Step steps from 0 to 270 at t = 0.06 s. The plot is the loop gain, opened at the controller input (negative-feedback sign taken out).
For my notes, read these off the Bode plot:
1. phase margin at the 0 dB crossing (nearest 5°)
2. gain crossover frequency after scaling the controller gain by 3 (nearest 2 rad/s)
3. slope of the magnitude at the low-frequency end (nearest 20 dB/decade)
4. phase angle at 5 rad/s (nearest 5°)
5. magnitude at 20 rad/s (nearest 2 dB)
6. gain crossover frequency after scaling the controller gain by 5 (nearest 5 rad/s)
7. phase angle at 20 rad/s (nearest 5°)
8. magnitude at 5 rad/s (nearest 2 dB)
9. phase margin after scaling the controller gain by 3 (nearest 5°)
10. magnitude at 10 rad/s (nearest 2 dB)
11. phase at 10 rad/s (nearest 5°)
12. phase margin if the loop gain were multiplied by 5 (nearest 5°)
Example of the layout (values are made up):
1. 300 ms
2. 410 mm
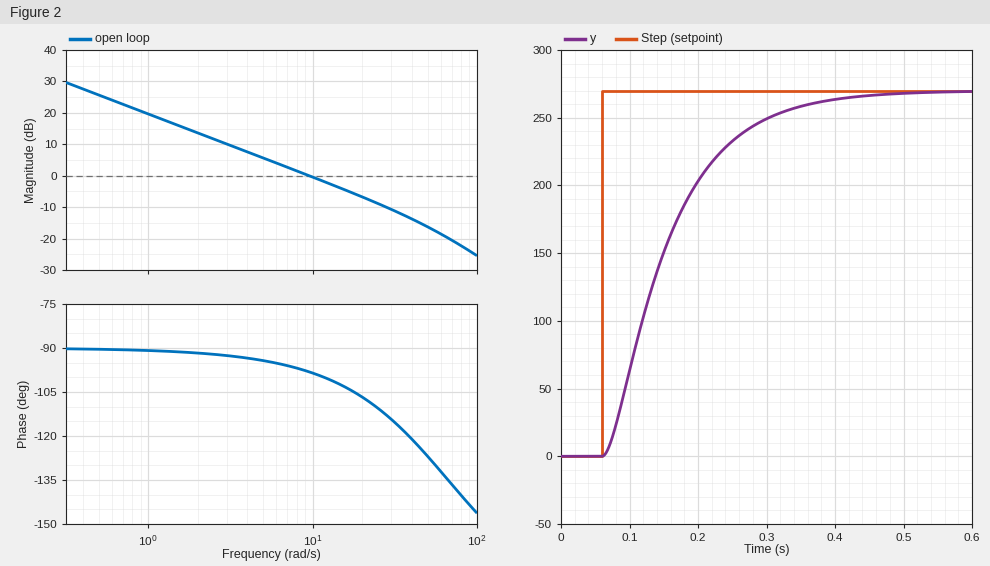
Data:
1. 80°
2. 26 rad/s
3. -20 dB/decade
4. -95°
5. -6 dB
6. 40 rad/s
7. -105°
8. 6 dB
9. 70°
10. 0 dB
11. -100°
12. 60°
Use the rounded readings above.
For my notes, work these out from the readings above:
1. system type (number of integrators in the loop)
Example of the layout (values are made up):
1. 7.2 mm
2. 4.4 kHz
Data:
1. 1
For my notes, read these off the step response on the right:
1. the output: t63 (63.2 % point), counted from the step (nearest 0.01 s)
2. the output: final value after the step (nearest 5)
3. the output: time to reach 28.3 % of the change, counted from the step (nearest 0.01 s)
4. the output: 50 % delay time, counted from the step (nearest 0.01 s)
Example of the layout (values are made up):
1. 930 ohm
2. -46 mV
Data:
1. 0.11 s
2. 270
3. 0.05 s
4. 0.08 s
